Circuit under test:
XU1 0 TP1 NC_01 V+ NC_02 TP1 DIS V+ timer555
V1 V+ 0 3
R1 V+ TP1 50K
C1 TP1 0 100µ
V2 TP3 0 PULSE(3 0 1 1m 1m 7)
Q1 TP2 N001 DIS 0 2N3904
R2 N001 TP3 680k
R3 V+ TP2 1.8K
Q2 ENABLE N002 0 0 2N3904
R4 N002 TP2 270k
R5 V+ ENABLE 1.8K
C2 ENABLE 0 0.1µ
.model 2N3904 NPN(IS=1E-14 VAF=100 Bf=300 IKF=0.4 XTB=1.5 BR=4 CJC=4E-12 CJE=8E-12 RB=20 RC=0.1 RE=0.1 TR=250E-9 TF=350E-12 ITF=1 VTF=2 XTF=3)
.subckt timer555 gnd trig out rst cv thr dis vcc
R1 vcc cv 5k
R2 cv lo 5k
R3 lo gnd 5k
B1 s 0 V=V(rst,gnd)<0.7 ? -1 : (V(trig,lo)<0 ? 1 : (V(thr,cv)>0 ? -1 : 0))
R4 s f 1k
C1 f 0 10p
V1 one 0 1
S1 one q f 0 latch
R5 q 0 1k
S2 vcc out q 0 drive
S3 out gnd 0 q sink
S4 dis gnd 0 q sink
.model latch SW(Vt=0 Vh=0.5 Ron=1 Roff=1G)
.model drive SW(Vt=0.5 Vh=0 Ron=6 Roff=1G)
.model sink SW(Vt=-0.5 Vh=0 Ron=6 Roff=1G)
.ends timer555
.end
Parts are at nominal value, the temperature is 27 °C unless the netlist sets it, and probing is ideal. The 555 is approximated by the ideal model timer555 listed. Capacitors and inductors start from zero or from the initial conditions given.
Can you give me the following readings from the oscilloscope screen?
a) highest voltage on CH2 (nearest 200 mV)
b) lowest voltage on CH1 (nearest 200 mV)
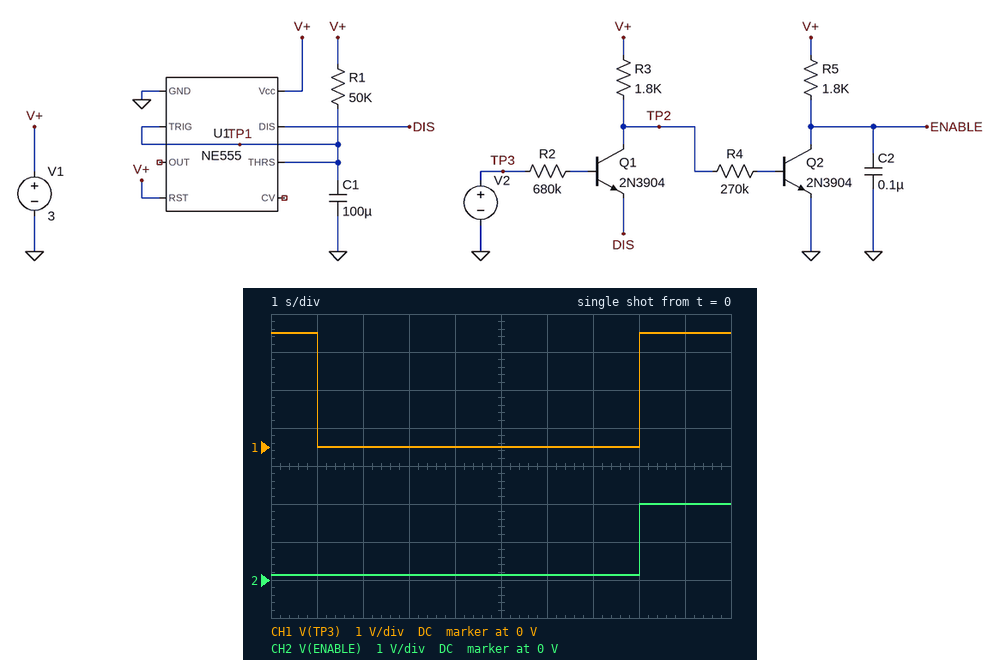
2.0 V
0 V
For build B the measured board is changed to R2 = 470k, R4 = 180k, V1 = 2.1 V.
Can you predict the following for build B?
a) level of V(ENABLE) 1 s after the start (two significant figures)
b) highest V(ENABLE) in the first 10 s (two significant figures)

110 mV
2.1 V
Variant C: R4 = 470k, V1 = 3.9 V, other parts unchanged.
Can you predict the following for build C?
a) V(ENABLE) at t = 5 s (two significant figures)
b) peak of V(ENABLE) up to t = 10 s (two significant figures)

260 mV
2.3 V
